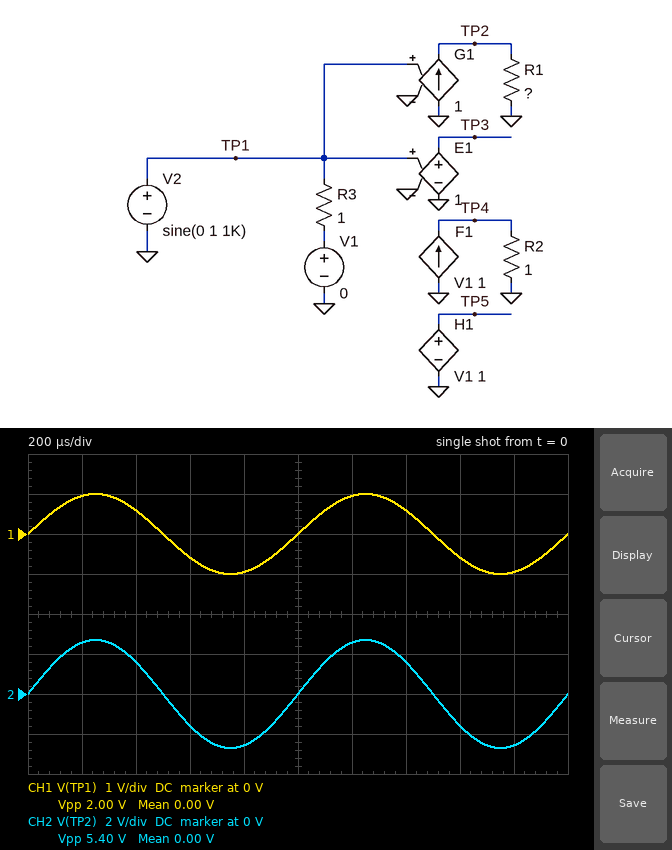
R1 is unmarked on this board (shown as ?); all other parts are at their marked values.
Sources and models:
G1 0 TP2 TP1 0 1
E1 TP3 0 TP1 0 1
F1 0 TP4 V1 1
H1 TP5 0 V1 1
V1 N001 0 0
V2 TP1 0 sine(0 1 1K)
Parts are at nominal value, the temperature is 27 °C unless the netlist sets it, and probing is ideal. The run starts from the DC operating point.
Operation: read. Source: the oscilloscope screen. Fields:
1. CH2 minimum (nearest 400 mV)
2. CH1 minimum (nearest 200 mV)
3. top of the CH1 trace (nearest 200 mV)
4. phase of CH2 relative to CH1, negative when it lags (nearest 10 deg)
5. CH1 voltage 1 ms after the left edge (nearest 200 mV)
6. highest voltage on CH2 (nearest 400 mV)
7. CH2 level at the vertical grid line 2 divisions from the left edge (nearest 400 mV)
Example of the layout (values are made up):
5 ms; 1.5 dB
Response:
-2.8 V; -1.0 V; 1.0 V; 0 deg; 0 V; 2.8 V; 1.6 V
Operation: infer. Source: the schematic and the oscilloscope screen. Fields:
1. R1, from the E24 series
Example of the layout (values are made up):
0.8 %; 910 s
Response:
2.7 Ω
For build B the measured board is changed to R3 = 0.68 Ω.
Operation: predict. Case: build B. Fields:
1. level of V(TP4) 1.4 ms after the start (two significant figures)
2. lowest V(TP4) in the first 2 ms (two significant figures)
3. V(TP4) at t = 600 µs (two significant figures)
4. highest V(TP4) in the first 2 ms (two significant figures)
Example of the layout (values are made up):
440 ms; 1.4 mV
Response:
860 mV; -1.5 V; -860 mV; 1.5 V
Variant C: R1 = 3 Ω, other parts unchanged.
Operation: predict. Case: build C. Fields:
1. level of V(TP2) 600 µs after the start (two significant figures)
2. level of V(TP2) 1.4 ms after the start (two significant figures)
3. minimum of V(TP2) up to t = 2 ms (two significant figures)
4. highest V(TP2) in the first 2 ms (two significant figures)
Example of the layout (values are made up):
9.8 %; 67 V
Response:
-1.8 V; 1.8 V; -3.0 V; 3.0 V
